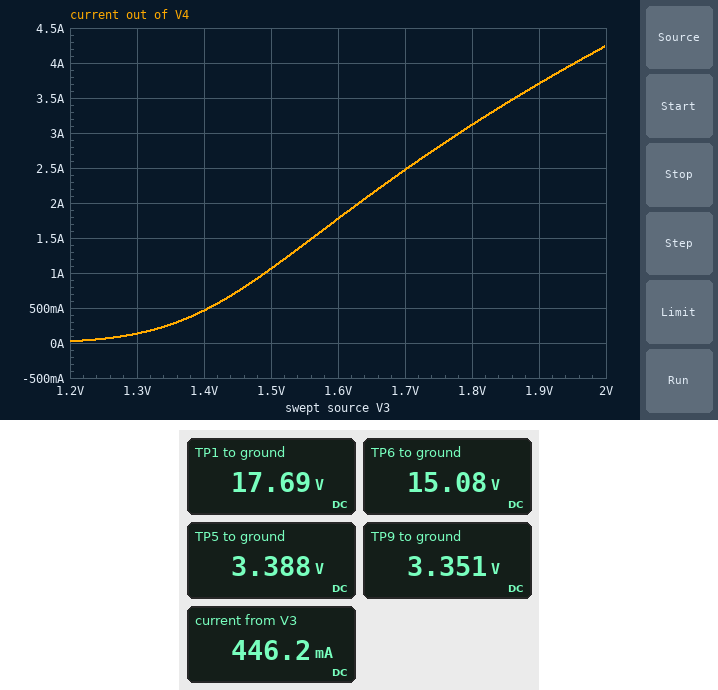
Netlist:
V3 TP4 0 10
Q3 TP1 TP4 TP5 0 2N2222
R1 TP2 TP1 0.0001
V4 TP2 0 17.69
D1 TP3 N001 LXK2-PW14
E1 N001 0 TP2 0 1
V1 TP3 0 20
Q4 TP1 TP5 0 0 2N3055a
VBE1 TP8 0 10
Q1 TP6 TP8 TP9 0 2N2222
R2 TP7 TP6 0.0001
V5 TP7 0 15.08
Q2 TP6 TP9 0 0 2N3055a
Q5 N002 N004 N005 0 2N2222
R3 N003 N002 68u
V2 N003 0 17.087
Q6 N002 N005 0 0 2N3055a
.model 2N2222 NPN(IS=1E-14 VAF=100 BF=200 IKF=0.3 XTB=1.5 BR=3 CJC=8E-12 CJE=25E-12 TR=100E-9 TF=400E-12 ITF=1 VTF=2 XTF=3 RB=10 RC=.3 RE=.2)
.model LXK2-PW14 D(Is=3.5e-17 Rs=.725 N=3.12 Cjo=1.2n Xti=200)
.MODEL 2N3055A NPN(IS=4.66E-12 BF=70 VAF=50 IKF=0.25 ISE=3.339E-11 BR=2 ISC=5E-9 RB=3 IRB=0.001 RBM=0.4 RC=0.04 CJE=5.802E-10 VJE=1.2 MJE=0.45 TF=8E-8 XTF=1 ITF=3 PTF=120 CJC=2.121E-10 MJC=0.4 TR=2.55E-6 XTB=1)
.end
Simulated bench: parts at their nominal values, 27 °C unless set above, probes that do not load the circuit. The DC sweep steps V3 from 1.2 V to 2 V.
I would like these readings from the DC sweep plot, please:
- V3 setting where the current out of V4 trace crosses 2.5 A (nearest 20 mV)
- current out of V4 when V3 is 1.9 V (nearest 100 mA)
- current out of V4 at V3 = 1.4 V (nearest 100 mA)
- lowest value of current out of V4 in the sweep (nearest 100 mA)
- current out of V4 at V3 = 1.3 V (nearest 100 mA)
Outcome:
1.70 V
3.7 A
500 mA
0 A
100 mA
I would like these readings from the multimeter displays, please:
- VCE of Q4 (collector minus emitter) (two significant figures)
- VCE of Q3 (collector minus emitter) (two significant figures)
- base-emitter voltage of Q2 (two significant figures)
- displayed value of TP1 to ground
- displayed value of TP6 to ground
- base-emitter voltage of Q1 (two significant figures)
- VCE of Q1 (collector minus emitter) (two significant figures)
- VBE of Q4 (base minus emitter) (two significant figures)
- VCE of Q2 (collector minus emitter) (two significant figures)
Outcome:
18 V
14 V
3.4 V
17.69 V
15.08 V
6.6 V
12 V
3.4 V
15 V
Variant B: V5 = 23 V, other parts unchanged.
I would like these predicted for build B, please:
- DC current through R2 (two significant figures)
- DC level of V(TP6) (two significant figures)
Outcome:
20 A
23 V
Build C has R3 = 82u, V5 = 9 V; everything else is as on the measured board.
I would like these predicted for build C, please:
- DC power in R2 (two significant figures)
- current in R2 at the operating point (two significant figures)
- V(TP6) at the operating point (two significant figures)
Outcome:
27 mW
17 A
9.0 V
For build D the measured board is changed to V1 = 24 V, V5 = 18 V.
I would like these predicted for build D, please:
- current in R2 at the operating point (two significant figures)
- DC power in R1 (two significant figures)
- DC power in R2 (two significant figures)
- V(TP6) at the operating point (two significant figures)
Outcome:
19 A
36 mW
36 mW
18 V
